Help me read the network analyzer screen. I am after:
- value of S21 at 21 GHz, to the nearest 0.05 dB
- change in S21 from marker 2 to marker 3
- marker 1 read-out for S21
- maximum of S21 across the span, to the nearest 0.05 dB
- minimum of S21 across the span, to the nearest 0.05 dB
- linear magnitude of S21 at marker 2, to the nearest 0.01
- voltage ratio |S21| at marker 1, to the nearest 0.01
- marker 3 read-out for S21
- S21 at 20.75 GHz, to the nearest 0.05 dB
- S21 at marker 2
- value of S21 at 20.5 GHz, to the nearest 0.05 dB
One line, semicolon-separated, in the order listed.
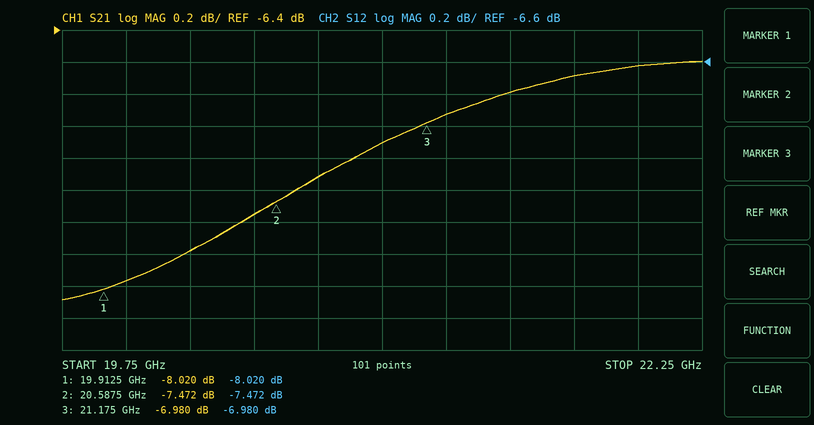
-7.10 dB; 0.492 dB; -8.020 dB; -6.60 dB; -8.10 dB; 0.42; 0.40; -6.980 dB; -7.30 dB; -7.472 dB; -7.55 dB
